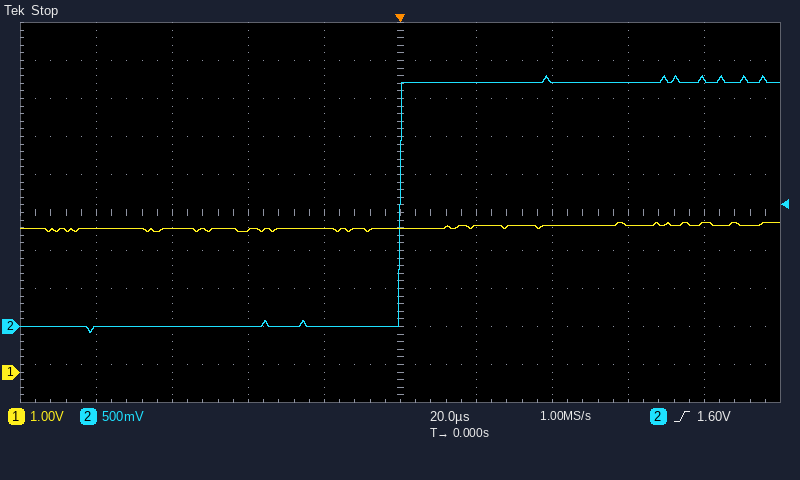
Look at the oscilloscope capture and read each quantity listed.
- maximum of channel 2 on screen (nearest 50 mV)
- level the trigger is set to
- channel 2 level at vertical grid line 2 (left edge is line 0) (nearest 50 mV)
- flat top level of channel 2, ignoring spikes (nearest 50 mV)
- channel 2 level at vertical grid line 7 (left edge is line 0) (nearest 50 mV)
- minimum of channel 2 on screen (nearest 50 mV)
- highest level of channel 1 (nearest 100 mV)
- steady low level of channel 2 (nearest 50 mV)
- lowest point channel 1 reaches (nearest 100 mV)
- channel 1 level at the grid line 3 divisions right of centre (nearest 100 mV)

3.30 V
1.60 V
0 mV
3.20 V
3.25 V
-100 mV
3.9 V
0 mV
3.7 V
3.9 V
